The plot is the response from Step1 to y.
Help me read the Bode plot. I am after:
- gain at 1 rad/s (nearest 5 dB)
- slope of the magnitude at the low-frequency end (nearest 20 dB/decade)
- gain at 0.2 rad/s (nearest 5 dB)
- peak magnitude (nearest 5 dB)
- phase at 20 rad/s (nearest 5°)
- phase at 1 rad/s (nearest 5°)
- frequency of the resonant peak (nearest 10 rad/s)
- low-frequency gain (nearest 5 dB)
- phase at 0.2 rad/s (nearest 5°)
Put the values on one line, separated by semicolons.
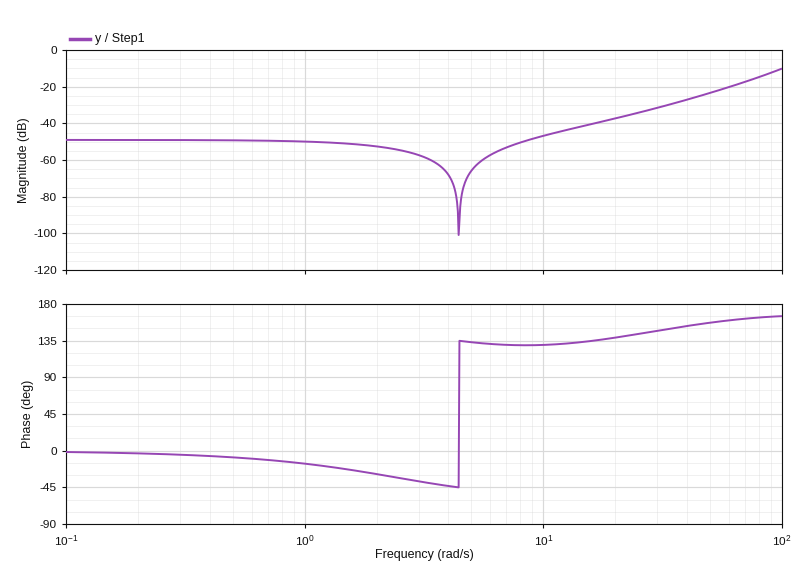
-50 dB; 0 dB/decade; -50 dB; -10 dB; 140°; -15°; 100 rad/s; -50 dB; -5°
